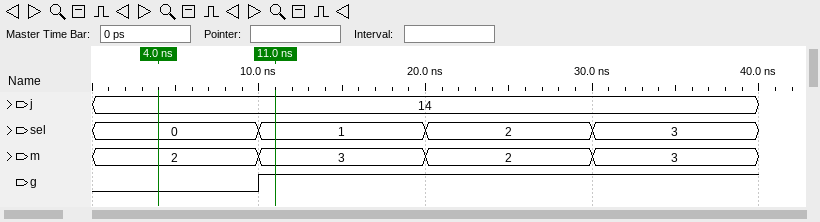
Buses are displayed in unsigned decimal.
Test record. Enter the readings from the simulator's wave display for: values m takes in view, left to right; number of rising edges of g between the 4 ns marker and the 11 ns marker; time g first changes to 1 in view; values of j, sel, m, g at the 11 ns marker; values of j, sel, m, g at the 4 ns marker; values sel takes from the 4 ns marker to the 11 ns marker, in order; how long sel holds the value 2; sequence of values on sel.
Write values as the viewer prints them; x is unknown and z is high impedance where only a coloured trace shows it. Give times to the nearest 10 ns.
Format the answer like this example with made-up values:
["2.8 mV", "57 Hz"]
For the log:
["2, 3, 2, 3", "1", "10 ns", "j=14, sel=1, m=3, g=1", "j=14, sel=0, m=2, g=0", "0, 1", "10 ns", "0, 1, 2, 3"]
